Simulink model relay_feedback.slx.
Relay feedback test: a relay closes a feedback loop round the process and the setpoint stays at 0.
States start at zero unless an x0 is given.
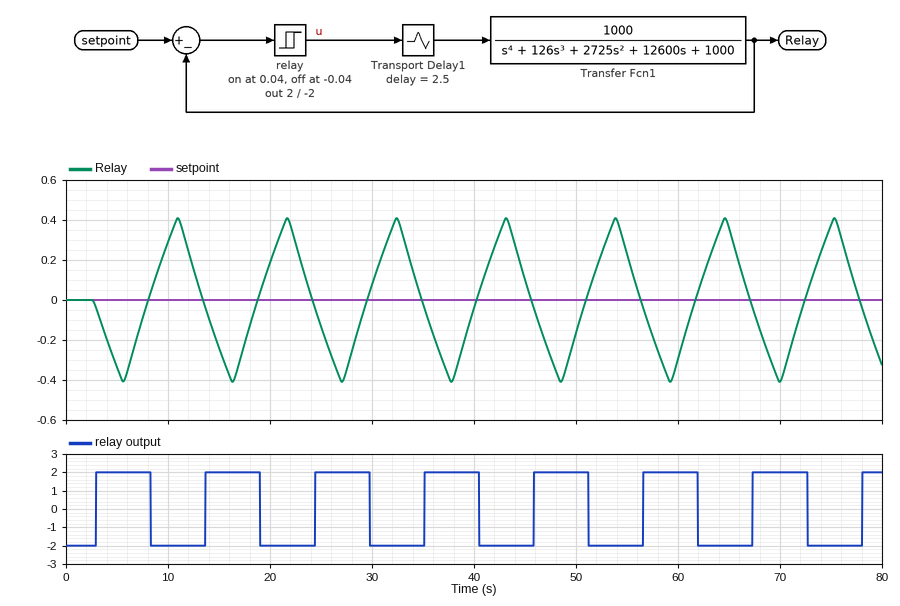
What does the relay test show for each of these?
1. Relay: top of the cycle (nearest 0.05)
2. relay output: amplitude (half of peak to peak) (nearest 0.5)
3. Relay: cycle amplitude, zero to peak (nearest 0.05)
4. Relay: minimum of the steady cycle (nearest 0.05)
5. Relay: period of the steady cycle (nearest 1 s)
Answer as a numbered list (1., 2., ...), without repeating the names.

1. 0.40
2. 2.0
3. 0.40
4. -0.40
5. 11 s
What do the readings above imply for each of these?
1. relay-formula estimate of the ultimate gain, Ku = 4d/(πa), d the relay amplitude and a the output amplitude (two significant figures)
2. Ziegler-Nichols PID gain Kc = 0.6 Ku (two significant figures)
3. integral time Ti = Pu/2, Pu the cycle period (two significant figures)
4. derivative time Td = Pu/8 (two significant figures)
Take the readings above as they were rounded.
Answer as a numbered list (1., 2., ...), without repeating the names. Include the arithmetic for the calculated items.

1. 4 × 2 / (π × 0.4) = 6.4
2. 0.6 × 6.4 = 3.8
3. 11 / 2 = 5.5 s
4. 11 / 8 = 1.4 s
